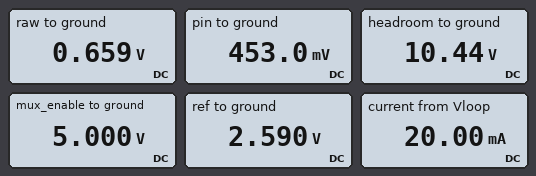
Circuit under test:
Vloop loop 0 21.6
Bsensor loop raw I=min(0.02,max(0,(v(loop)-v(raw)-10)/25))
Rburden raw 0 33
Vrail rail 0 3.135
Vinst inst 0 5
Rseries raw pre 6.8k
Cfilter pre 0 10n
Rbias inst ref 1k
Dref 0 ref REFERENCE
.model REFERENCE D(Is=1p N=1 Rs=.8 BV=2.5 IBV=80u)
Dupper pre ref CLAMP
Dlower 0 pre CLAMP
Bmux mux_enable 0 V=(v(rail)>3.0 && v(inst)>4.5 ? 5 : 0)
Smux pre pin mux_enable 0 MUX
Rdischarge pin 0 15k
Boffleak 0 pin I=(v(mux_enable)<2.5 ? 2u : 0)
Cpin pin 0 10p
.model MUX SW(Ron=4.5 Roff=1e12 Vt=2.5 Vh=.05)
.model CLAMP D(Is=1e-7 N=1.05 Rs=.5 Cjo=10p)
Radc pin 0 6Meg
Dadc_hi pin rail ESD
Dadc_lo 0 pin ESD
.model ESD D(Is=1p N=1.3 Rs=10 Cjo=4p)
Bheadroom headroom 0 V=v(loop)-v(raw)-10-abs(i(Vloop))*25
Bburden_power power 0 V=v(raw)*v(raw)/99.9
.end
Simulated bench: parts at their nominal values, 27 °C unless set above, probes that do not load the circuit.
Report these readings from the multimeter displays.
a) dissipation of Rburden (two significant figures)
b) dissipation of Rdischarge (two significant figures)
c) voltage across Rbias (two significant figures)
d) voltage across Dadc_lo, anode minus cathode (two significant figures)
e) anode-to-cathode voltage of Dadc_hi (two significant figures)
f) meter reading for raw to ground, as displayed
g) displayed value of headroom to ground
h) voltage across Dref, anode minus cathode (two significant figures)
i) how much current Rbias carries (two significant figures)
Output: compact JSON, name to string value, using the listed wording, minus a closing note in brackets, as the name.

{"dissipation of Rburden": "13 mW", "dissipation of Rdischarge": "14 µW", "voltage across Rbias": "2.4 V", "voltage across Dadc_lo, anode minus cathode": "-450 mV", "anode-to-cathode voltage of Dadc_hi": "-2.7 V", "meter reading for raw to ground, as displayed": "0.659 V", "displayed value of headroom to ground": "10.44 V", "voltage across Dref, anode minus cathode": "-2.6 V", "how much current Rbias carries": "2.4 mA"}
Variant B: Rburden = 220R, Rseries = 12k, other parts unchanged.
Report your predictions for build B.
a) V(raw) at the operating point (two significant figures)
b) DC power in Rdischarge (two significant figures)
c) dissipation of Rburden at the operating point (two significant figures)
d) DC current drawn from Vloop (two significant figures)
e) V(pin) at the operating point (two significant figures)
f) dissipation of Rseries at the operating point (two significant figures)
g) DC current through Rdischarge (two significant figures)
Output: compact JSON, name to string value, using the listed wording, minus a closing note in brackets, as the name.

{"V(raw) at the operating point": "4.4 V", "DC power in Rdischarge": "390 µW", "dissipation of Rburden at the operating point": "87 mW", "DC current drawn from Vloop": "20 mA", "V(pin) at the operating point": "2.4 V", "dissipation of Rseries at the operating point": "310 µW", "DC current through Rdischarge": "160 µA"}
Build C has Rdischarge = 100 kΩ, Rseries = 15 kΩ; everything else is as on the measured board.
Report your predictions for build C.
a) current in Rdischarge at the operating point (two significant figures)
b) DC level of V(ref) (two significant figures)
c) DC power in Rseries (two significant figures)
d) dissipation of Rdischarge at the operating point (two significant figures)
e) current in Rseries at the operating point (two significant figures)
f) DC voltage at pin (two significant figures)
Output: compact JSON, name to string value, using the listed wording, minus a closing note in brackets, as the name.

{"current in Rdischarge at the operating point": "5.7 µA", "DC level of V(ref)": "2.6 V", "DC power in Rseries": "510 nW", "dissipation of Rdischarge at the operating point": "3.3 µW", "current in Rseries at the operating point": "5.8 µA", "DC voltage at pin": "570 mV"}
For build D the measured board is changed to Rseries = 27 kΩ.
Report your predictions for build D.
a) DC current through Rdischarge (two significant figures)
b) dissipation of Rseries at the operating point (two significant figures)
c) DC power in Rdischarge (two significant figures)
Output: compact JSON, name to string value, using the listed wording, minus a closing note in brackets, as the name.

{"DC current through Rdischarge": "16 µA", "dissipation of Rseries at the operating point": "6.7 µW", "DC power in Rdischarge": "3.7 µW"}
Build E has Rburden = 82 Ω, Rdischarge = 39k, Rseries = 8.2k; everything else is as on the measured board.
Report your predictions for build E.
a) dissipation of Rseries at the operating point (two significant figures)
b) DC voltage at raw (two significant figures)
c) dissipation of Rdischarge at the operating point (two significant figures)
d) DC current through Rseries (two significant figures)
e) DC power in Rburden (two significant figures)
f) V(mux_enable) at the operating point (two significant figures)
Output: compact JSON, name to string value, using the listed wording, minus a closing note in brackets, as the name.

{"dissipation of Rseries at the operating point": "10 µW", "DC voltage at raw": "1.6 V", "dissipation of Rdischarge at the operating point": "47 µW", "DC current through Rseries": "35 µA", "DC power in Rburden": "33 mW", "V(mux_enable) at the operating point": "5.0 V"}
